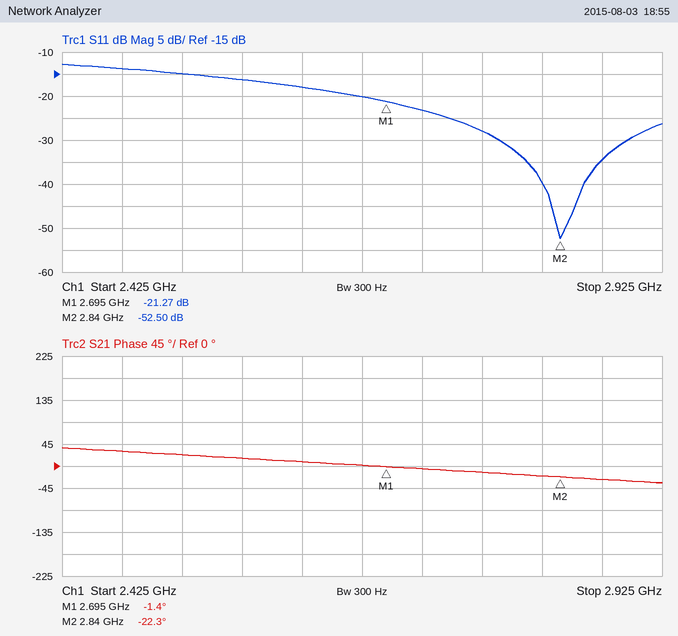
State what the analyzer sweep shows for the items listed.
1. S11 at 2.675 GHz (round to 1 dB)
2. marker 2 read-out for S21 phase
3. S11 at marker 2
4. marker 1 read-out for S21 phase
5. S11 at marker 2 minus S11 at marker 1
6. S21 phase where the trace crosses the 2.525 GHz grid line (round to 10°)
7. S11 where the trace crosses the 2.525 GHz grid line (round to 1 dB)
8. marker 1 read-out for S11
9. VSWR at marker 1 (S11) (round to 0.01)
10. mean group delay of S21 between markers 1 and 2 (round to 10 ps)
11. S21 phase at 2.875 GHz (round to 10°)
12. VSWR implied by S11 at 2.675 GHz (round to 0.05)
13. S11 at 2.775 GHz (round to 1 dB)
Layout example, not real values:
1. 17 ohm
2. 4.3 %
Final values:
1. -20 dB
2. -22.3°
3. -52.50 dB
4. -1.4°
5. -31.23 dB
6. 20°
7. -15 dB
8. -21.27 dB
9. 1.19
10. 400 ps
11. -30°
12. 1.20
13. -28 dB
